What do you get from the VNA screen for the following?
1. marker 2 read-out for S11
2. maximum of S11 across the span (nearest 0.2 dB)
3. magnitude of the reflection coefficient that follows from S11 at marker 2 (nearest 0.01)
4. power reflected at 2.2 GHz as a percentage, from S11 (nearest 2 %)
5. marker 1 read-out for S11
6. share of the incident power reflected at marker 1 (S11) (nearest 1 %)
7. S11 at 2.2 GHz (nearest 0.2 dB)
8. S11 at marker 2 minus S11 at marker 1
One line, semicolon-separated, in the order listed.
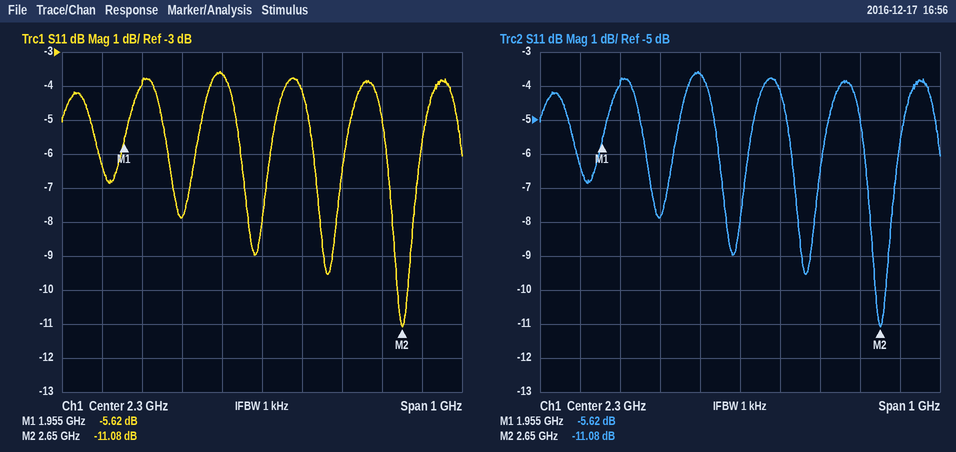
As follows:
-11.08 dB; -3.6 dB; 0.28; 44 %; -5.62 dB; 27 %; -3.6 dB; -5.46 dB
